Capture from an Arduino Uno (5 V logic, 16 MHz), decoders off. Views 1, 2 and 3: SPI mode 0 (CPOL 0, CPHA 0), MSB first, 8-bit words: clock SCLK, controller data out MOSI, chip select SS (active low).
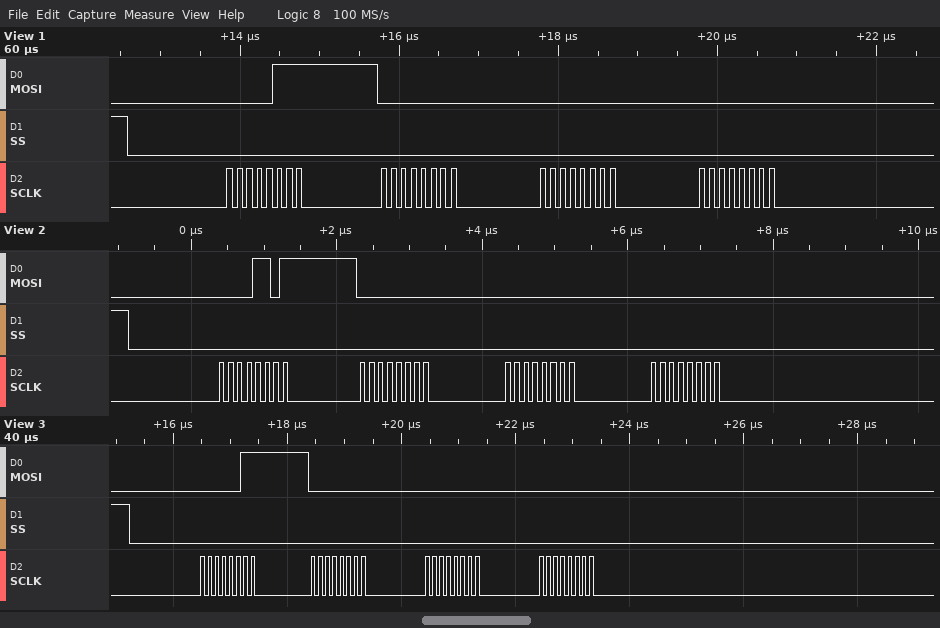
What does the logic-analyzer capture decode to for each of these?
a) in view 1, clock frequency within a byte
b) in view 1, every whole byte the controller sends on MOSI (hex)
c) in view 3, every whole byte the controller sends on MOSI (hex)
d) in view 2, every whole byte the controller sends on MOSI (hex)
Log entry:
8 MHz
07 00 00 00
03 00 00 00
0D 00 00 00
